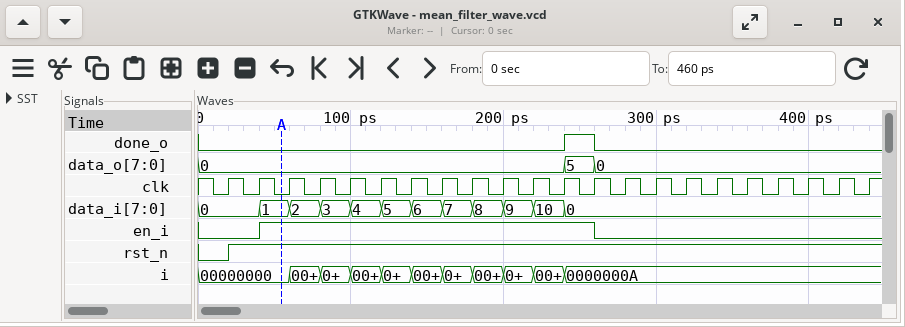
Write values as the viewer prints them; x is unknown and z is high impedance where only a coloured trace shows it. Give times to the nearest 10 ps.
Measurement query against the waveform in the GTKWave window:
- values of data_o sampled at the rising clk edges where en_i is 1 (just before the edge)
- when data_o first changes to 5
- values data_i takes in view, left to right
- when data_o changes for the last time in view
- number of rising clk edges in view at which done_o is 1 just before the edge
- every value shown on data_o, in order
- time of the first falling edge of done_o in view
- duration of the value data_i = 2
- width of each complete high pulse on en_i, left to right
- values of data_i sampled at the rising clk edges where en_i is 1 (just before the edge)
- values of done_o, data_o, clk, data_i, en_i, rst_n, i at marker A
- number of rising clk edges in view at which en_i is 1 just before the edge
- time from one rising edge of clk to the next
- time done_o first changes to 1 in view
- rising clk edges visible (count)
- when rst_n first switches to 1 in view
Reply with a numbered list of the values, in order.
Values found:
1. 0, 0, 0, 0, 0, 0, 0, 0, 0, 0, 5
2. 240 ps
3. 0, 1, 2, 3, 4, 5, 6, 7, 8, 9, 10, 0
4. 260 ps
5. 1
6. 0, 5, 0
7. 260 ps
8. 20 ps
9. 220 ps
10. 1, 2, 3, 4, 5, 6, 7, 8, 9, 10, 0
11. done_o=0, data_o=0, clk=0, data_i=1, en_i=1, rst_n=1, i=00000000
12. 11
13. 20 ps
14. 240 ps
15. 22
16. 20 ps
